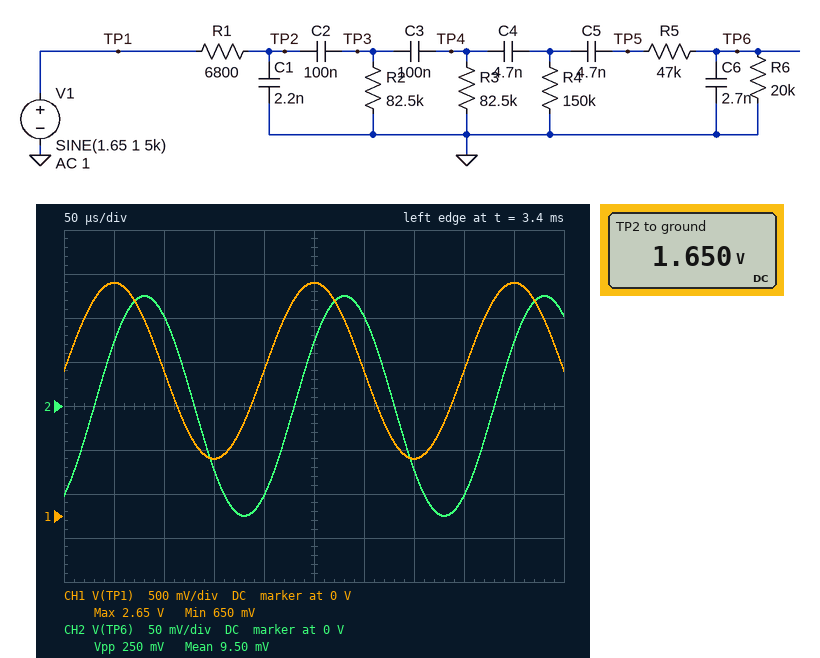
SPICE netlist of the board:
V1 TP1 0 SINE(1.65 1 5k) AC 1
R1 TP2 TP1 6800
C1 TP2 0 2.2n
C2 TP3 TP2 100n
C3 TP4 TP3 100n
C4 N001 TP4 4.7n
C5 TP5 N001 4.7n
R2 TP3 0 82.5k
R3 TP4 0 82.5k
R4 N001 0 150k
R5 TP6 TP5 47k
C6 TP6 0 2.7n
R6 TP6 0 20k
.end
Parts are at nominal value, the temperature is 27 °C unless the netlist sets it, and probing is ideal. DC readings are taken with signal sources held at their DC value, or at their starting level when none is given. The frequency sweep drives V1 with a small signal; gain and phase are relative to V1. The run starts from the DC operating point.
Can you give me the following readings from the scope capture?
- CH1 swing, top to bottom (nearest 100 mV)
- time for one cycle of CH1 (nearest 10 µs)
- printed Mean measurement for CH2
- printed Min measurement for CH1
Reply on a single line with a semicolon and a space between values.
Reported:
2.0 V; 200 µs; 9.50 mV; 650 mV
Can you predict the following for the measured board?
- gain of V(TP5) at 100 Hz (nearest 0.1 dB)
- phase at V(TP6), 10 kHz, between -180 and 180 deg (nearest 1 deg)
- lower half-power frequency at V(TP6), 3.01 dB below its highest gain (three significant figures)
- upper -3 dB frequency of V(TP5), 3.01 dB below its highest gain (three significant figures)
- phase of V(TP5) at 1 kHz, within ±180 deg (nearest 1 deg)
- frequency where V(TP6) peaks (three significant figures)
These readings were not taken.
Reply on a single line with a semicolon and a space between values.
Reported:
-26.8 dB; -94 deg; 696 Hz; 17.4 kHz; 49 deg; 2.00 kHz
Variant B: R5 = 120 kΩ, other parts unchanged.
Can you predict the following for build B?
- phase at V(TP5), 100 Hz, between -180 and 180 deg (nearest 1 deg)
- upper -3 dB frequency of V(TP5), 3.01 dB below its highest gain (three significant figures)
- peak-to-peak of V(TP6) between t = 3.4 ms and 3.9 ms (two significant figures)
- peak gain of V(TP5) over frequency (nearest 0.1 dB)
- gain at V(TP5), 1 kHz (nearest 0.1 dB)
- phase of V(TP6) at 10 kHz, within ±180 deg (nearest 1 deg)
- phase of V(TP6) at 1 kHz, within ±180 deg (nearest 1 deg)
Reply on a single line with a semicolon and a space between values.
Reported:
148 deg; 15.0 kHz; 120 mV; -2.6 dB; -3.6 dB; -103 deg; 18 deg
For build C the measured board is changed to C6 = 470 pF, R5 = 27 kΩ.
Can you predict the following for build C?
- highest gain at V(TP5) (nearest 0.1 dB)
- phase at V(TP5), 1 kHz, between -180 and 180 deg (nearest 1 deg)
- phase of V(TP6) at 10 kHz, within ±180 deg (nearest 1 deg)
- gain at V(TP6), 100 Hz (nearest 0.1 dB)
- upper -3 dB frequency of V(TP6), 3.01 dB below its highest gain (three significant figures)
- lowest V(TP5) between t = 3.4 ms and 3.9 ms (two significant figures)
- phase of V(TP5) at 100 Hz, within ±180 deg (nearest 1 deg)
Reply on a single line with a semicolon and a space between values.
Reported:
-3.9 dB; 58 deg; -45 deg; -37.1 dB; 14.0 kHz; -640 mV; 159 deg
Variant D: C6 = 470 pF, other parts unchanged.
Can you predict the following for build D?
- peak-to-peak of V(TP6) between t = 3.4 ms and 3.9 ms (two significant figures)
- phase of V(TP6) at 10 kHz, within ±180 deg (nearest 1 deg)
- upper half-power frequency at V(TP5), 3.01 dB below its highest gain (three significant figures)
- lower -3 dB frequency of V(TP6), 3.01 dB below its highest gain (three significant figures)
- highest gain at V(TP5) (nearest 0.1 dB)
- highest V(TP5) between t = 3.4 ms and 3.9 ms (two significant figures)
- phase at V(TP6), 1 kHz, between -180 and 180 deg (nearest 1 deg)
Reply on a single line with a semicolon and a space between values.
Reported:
400 mV; -51 deg; 15.9 kHz; 903 Hz; -3.2 dB; 680 mV; 48 deg
